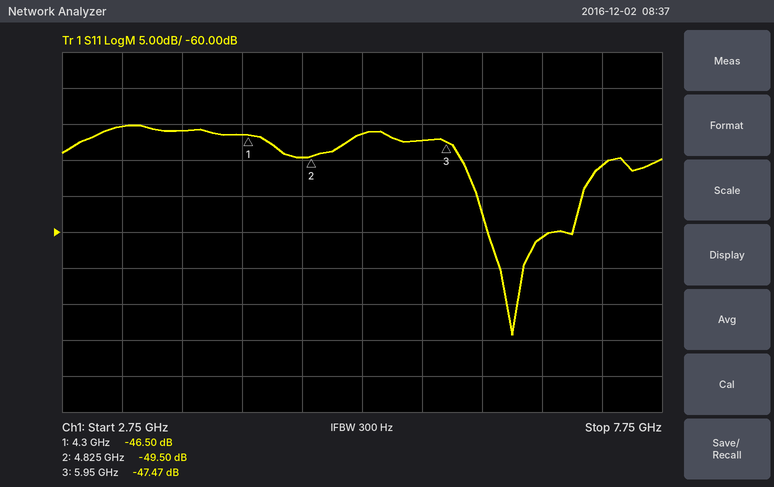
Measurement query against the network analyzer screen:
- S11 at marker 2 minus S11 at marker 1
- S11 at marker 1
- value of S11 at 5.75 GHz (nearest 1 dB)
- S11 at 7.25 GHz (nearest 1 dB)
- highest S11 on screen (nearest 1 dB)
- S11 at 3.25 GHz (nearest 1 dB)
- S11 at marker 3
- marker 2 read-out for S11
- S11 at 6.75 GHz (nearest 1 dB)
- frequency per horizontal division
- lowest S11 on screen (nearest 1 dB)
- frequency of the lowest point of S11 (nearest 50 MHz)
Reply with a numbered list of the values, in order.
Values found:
1. -3.00 dB
2. -46.50 dB
3. -47 dB
4. -51 dB
5. -45 dB
6. -45 dB
7. -47.47 dB
8. -49.50 dB
9. -61 dB
10. 500 MHz
11. -74 dB
12. 6.50 GHz
